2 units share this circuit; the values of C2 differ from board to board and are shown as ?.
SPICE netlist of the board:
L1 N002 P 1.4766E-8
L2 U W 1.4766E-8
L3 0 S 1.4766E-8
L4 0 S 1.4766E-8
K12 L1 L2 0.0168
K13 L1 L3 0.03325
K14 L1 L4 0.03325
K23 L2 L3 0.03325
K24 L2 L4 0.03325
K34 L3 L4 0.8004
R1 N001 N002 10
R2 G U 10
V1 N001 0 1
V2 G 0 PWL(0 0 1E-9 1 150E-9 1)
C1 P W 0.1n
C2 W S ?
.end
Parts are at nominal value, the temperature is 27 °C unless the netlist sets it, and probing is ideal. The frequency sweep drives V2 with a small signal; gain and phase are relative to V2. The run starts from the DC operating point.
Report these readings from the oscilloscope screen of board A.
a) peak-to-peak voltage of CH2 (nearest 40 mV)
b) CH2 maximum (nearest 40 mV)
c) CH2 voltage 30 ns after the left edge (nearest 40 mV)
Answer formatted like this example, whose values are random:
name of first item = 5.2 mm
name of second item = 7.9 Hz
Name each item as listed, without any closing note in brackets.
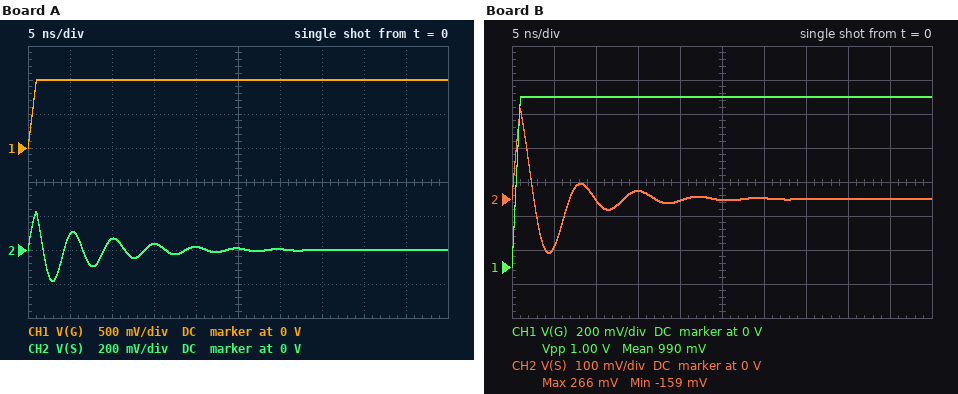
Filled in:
peak-to-peak voltage of CH2 = 400 mV
CH2 maximum = 240 mV
CH2 voltage 30 ns after the left edge = 0 V
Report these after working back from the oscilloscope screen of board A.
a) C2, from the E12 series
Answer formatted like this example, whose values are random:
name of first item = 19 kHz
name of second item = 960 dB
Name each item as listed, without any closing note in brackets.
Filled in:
C2, from the E12 series = 33 pF
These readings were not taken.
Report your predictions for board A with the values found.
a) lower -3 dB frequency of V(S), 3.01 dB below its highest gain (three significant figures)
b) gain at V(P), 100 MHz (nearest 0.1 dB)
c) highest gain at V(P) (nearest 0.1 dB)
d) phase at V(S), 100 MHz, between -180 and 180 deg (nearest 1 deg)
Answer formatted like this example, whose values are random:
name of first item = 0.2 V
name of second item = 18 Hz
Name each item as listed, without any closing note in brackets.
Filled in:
lower -3 dB frequency of V(S), 3.01 dB below its highest gain = 191 MHz
gain at V(P), 100 MHz = -3.6 dB
highest gain at V(P) = -0.8 dB
phase at V(S), 100 MHz, between -180 and 180 deg = 128 deg
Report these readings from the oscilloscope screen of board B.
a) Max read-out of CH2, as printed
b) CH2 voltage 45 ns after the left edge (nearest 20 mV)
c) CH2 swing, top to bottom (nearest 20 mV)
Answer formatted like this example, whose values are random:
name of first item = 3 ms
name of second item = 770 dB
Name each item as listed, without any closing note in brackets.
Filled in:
Max read-out of CH2, as printed = 266 mV
CH2 voltage 45 ns after the left edge = 0 V
CH2 swing, top to bottom = 420 mV
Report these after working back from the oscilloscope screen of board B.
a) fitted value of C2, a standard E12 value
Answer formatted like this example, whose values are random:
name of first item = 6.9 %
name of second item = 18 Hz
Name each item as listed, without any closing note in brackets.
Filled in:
fitted value of C2, a standard E12 value = 82 pF
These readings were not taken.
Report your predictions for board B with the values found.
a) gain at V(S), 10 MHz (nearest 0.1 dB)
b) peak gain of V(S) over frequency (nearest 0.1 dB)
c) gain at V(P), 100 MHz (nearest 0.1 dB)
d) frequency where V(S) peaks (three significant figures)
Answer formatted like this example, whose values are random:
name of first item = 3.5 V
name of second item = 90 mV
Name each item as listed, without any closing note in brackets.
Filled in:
gain at V(S), 10 MHz = -47.6 dB
peak gain of V(S) over frequency = -2.2 dB
gain at V(P), 100 MHz = -5.1 dB
frequency where V(S) peaks = 145 MHz
